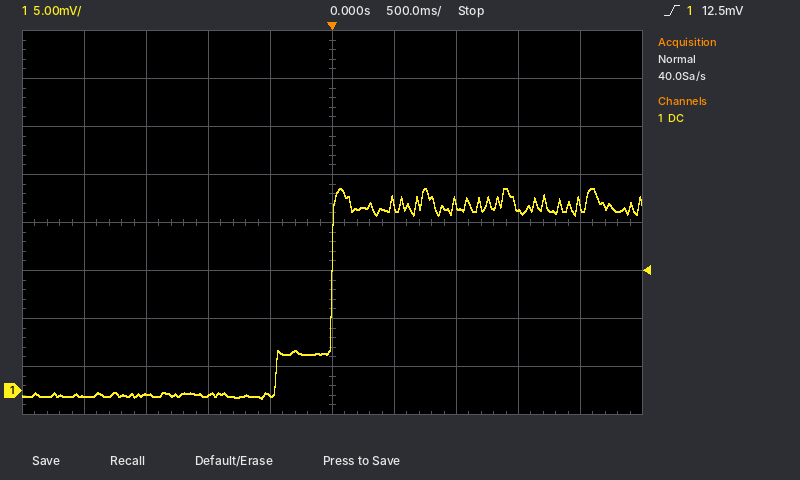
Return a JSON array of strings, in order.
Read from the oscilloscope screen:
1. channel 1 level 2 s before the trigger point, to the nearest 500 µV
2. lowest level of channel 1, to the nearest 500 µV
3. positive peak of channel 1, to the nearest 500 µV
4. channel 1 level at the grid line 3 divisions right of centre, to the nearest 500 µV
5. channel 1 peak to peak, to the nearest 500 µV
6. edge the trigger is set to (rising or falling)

["-500 µV", "-1.0 mV", "21.0 mV", "19.0 mV", "22.0 mV", "rising"]
